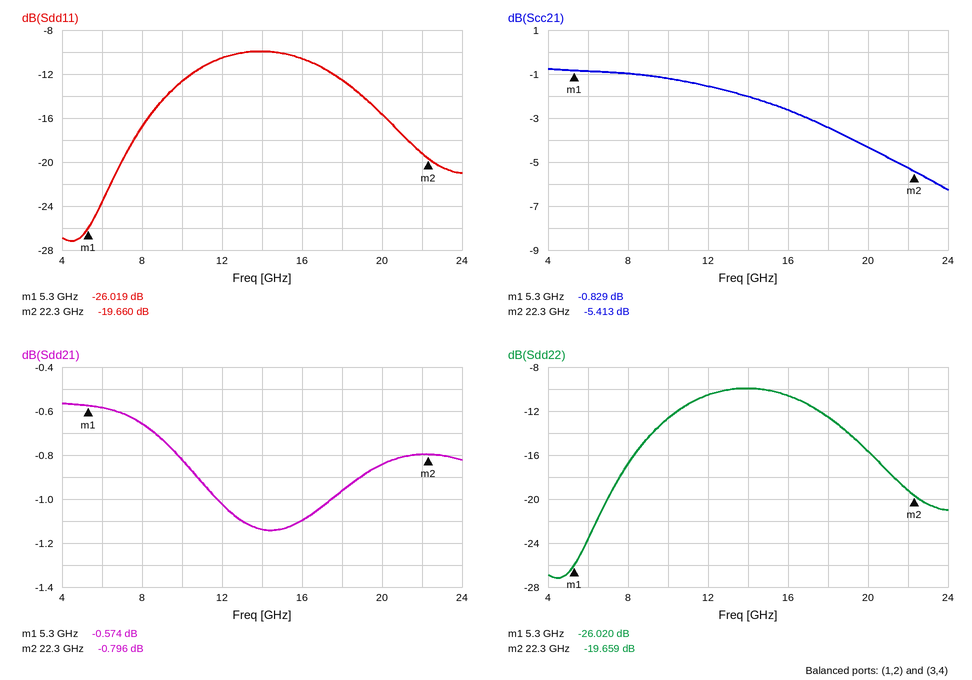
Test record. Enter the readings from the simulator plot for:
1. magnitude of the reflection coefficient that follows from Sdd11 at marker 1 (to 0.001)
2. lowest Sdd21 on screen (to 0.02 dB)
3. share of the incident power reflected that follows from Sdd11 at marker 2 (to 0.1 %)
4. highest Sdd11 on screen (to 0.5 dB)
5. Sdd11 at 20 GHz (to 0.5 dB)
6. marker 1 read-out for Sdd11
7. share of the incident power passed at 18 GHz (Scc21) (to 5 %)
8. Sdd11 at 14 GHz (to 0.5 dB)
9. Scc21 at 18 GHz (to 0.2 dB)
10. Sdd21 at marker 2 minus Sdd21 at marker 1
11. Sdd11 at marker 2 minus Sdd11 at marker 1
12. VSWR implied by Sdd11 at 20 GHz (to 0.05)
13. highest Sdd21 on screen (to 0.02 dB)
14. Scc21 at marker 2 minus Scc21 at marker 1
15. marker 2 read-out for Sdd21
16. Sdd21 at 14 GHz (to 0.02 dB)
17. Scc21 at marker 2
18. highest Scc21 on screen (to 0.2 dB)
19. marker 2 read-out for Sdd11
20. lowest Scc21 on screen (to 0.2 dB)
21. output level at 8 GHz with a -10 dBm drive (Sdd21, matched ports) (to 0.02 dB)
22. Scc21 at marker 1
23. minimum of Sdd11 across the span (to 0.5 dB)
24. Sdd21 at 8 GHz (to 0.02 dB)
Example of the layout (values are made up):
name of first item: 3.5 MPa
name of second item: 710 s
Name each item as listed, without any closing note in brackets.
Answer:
magnitude of the reflection coefficient that follows from Sdd11 at marker 1: 0.050
lowest Sdd21 on screen: -1.14 dB
share of the incident power reflected that follows from Sdd11 at marker 2: 1.1 %
highest Sdd11 on screen: -10.0 dB
Sdd11 at 20 GHz: -15.5 dB
marker 1 read-out for Sdd11: -26.019 dB
share of the incident power passed at 18 GHz (Scc21): 45 %
Sdd11 at 14 GHz: -10.0 dB
Scc21 at 18 GHz: -3.4 dB
Sdd21 at marker 2 minus Sdd21 at marker 1: -0.222 dB
Sdd11 at marker 2 minus Sdd11 at marker 1: 6.359 dB
VSWR implied by Sdd11 at 20 GHz: 1.40
highest Sdd21 on screen: -0.56 dB
Scc21 at marker 2 minus Scc21 at marker 1: -4.584 dB
marker 2 read-out for Sdd21: -0.796 dB
Sdd21 at 14 GHz: -1.14 dB
Scc21 at marker 2: -5.413 dB
highest Scc21 on screen: -0.8 dB
marker 2 read-out for Sdd11: -19.660 dB
lowest Scc21 on screen: -6.2 dB
output level at 8 GHz with a -10 dBm drive (Sdd21, matched ports): -10.66 dBm
Scc21 at marker 1: -0.829 dB
minimum of Sdd11 across the span: -27.0 dB
Sdd21 at 8 GHz: -0.66 dB
